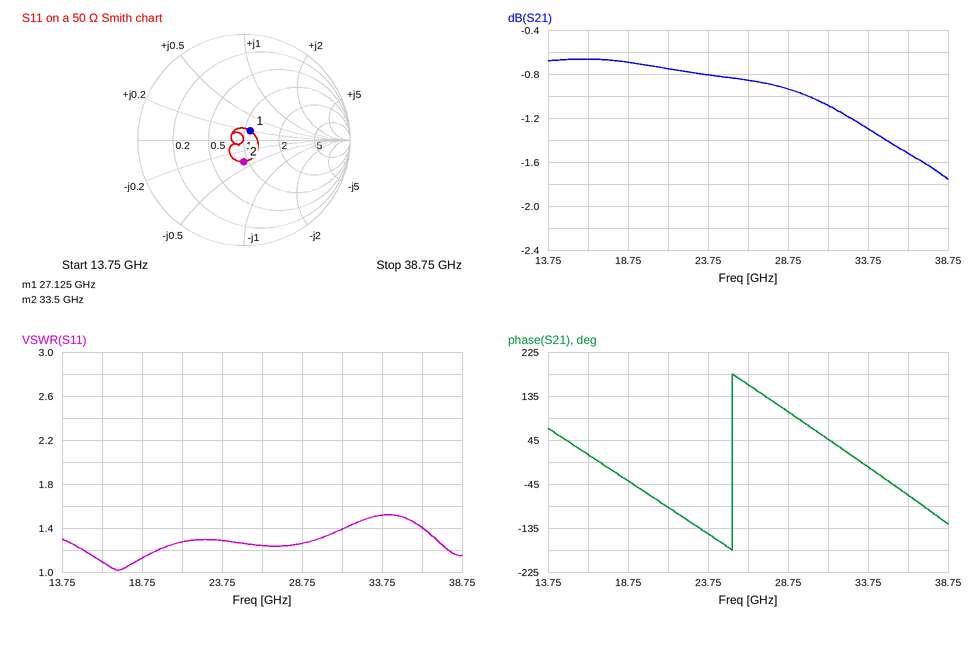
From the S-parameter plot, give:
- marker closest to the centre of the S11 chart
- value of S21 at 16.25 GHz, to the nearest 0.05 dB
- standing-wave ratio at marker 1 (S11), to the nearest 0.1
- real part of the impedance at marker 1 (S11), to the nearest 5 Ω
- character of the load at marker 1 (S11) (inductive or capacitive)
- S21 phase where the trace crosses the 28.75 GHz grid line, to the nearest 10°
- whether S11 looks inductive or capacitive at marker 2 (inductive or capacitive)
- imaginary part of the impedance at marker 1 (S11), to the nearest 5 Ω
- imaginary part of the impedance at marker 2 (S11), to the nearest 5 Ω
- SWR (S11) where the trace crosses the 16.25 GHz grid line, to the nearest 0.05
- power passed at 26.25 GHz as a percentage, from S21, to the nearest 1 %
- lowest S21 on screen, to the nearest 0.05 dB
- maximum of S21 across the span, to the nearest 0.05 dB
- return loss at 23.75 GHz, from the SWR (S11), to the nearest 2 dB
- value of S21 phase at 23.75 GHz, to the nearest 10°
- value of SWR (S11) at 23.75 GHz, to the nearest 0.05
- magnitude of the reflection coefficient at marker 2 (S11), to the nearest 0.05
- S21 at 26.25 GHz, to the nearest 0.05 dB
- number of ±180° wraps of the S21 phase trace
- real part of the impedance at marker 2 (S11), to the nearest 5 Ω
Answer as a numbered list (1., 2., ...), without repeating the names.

1. marker 1
2. -0.65 dB
3. 1.2
4. 55 Ω
5. inductive
6. 100°
7. capacitive
8. +10 Ω
9. -20 Ω
10. 1.10
11. 82 %
12. -1.75 dB
13. -0.65 dB
14. 18 dB
15. -150°
16. 1.30
17. 0.20
18. -0.85 dB
19. 1
20. 45 Ω
